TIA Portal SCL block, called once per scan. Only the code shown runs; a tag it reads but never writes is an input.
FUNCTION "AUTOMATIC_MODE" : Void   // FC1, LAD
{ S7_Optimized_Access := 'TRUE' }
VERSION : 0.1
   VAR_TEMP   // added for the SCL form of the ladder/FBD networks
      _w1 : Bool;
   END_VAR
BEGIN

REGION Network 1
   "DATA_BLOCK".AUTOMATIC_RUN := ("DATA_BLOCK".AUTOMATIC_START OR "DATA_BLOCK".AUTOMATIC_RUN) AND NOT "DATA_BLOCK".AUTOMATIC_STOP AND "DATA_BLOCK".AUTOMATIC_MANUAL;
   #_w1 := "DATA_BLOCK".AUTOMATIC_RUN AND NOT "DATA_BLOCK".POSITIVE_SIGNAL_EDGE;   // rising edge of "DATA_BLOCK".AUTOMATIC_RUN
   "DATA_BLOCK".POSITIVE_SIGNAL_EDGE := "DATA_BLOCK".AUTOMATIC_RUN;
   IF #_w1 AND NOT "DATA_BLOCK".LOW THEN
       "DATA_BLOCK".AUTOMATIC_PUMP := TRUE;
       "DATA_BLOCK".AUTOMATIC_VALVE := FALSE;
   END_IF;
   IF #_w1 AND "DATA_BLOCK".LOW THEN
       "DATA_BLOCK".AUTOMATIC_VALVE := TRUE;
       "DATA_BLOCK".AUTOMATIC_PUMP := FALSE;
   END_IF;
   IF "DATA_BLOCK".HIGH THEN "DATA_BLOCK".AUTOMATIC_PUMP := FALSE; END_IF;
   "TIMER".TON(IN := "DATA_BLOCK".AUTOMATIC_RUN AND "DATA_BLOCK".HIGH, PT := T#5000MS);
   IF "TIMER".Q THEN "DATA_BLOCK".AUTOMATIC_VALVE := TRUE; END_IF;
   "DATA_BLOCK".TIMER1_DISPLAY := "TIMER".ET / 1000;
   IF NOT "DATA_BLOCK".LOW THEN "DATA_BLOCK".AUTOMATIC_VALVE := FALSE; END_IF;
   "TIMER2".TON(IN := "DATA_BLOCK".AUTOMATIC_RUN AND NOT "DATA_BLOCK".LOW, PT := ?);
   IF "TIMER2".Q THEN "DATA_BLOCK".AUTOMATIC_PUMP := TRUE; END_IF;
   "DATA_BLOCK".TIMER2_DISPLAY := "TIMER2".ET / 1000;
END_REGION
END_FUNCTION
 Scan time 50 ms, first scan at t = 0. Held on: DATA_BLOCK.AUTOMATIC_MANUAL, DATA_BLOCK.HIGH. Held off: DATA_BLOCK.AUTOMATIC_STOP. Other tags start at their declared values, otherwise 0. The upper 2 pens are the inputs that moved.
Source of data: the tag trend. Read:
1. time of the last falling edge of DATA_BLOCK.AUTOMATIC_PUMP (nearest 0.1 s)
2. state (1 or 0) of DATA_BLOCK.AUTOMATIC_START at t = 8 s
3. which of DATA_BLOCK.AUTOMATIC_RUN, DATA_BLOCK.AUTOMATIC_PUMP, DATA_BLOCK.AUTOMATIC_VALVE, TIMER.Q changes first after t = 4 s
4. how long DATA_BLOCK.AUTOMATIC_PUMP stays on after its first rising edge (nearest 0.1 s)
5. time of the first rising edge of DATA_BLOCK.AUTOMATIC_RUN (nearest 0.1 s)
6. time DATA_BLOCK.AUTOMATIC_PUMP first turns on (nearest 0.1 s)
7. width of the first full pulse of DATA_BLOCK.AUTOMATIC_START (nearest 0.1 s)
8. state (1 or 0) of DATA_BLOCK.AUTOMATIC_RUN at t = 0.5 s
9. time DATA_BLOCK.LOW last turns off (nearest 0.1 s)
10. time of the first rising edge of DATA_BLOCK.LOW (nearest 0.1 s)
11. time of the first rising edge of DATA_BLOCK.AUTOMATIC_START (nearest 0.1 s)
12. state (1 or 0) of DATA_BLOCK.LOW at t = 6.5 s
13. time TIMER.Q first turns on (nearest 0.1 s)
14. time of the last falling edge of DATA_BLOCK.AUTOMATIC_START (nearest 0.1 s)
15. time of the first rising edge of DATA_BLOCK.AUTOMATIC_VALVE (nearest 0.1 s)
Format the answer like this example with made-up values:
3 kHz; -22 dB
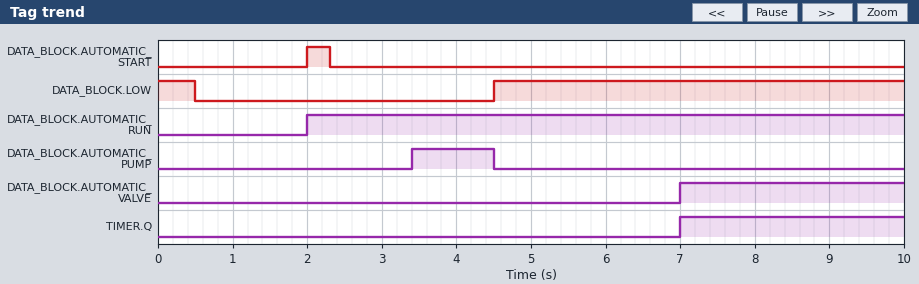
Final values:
4.5 s; 0; DATA_BLOCK.AUTOMATIC_PUMP; 1.1 s; 2.0 s; 3.4 s; 0.3 s; 0; 0.5 s; 4.5 s; 2.0 s; 1; 7.0 s; 2.3 s; 7.0 s
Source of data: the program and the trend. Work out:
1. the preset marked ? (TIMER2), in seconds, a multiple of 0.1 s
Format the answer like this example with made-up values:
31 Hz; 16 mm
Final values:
1.4 s
